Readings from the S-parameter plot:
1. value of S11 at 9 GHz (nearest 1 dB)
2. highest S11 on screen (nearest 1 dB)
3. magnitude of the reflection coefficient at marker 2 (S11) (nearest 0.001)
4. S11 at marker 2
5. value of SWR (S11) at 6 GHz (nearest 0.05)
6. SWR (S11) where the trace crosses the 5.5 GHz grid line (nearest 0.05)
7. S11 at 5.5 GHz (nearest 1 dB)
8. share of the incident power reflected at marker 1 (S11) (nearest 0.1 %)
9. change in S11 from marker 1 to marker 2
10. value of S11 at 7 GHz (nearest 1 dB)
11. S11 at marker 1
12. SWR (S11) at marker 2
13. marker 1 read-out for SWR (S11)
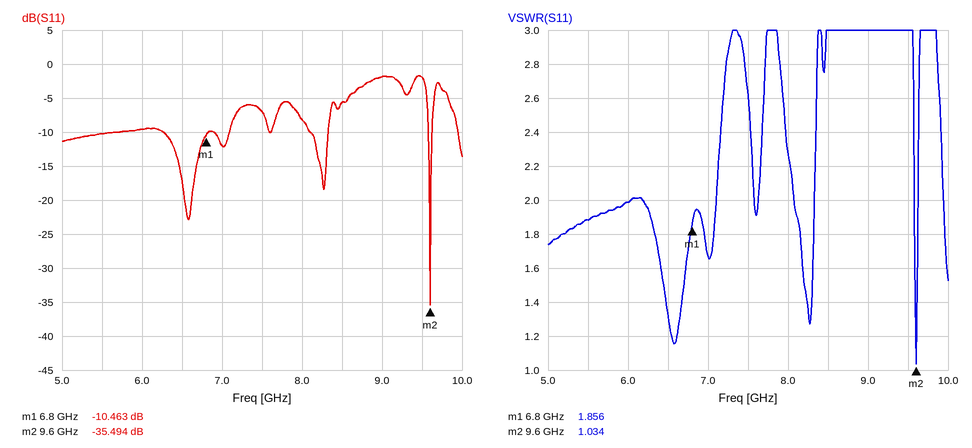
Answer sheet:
-2 dB
-2 dB
0.017
-35.494 dB
2.00
1.90
-10 dB
9.0 %
-25.031 dB
-12 dB
-10.463 dB
1.034
1.856
